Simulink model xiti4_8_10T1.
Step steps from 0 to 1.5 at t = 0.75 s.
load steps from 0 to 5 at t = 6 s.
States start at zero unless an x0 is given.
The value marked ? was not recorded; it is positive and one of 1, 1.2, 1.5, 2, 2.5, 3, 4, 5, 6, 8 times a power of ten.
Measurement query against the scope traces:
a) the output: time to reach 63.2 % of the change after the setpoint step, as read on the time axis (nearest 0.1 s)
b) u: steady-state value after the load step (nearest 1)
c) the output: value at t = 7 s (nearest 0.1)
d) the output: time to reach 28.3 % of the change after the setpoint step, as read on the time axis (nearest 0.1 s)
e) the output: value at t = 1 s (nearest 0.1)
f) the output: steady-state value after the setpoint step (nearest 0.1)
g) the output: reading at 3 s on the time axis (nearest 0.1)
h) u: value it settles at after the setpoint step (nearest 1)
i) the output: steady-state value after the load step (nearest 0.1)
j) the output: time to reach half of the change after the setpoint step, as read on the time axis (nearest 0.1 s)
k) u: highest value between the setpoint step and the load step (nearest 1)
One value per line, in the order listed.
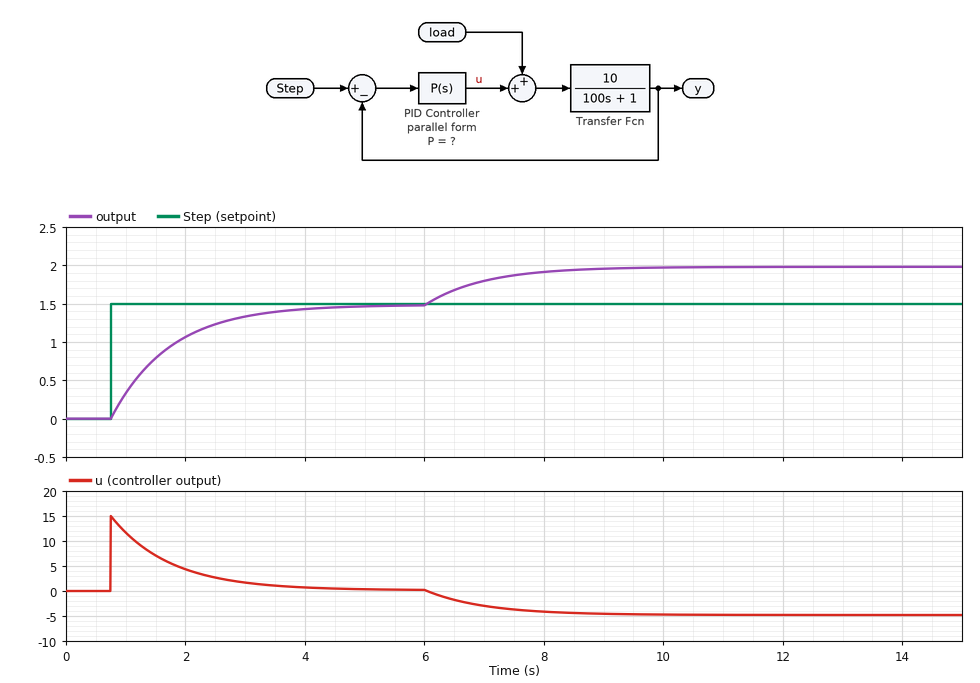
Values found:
1.7 s
-5
1.8
1.1 s
0.3
1.5
1.3
0
2.0
1.4 s
15
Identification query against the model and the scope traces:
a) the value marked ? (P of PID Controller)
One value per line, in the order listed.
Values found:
10
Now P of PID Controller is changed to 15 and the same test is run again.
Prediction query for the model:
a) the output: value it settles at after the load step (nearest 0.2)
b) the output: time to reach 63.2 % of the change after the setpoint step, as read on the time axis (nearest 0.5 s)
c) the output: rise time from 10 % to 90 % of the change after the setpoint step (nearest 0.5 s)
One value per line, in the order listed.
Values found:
1.8
1.5 s
1.5 s
